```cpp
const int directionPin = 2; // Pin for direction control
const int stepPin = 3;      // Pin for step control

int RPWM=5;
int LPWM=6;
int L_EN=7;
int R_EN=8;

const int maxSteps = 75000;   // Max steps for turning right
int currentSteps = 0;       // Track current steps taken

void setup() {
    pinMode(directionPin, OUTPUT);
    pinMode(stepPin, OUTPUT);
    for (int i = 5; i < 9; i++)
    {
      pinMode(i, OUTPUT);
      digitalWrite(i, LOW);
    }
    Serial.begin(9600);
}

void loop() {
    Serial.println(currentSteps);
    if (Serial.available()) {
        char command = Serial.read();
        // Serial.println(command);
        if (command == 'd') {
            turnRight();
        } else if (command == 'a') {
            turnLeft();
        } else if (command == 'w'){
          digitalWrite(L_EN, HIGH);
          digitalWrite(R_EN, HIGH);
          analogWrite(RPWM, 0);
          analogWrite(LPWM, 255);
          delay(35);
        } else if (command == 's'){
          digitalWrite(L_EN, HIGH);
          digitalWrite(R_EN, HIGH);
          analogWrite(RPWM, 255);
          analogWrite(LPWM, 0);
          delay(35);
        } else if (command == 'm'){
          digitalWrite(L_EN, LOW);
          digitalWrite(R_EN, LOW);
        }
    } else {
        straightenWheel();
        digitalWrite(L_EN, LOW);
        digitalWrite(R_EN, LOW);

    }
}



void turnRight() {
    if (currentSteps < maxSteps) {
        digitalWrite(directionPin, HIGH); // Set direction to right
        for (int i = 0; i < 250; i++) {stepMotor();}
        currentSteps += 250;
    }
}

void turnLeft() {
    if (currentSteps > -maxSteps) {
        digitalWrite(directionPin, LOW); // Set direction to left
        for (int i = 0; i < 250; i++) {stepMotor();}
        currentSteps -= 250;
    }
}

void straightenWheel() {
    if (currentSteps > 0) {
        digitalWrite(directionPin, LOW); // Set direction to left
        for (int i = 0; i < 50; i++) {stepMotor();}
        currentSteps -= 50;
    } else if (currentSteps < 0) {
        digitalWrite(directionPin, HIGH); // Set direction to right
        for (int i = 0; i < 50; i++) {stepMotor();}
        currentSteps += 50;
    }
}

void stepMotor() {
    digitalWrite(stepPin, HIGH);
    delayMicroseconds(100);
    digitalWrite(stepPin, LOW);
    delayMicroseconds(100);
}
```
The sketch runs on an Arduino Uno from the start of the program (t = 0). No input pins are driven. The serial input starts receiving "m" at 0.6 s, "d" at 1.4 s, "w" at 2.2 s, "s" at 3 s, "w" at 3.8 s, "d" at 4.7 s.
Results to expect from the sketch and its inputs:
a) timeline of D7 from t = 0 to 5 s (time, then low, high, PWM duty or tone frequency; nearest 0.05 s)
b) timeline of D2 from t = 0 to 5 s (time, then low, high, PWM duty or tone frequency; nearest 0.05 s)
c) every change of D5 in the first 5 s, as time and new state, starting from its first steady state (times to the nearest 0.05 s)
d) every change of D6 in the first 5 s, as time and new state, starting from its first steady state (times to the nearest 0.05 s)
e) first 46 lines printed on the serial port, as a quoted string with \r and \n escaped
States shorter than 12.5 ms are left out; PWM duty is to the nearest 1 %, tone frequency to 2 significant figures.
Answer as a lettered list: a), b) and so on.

a) 0 s low; 2.2 s high; 2.25 s low; 3 s high; 3.05 s low; 3.8 s high; 3.85 s low
b) 0 s low; 1.4 s high; 1.45 s low; 4.7 s high; 4.75 s low
c) 0 s low; 3 s high; 3.8 s low
d) 0 s low; 2.2 s high; 3 s low; 3.8 s high
e) "0\r\n0\r\n0\r\n0\r\n0\r\n0\r\n0\r\n0\r\n0\r\n0\r\n0\r\n0\r\n0\r\n0\r\n0\r\n0\r\n0\r\n0\r\n0\r\n0\r\n0\r\n0\r\n0\r\n0\r\n0\r\n0\r\n0\r\n0\r\n0\r\n0\r\n0\r\n0\r\n0\r\n0\r\n0\r\n0\r\n0\r\n0\r\n0\r\n0\r\n0\r\n0\r\n0\r\n0\r\n0\r\n0\r\n"
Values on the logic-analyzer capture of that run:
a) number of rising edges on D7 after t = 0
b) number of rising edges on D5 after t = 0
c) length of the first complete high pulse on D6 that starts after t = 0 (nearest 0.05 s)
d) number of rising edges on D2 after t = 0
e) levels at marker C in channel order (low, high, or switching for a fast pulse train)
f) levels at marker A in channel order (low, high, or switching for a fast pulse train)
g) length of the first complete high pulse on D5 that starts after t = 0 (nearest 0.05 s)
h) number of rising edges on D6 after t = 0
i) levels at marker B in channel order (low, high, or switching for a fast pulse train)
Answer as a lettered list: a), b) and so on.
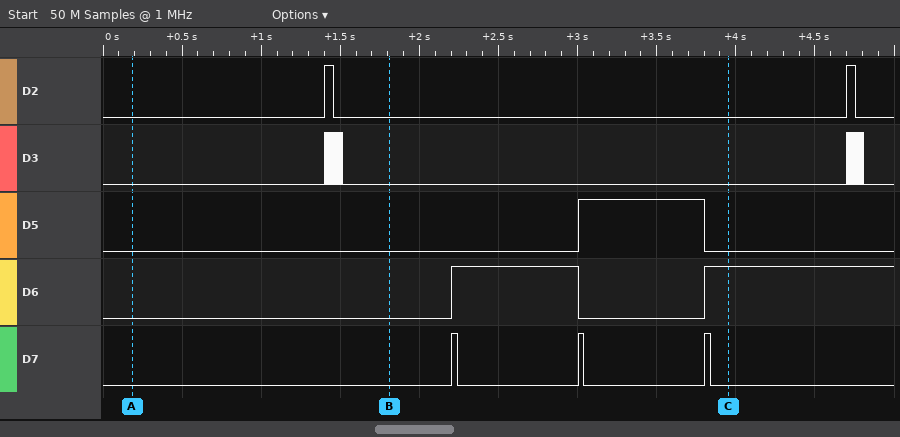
a) 3
b) 1
c) 0.80 s
d) 2
e) D2 low, D3 low, D5 low, D6 high, D7 low
f) D2 low, D3 low, D5 low, D6 low, D7 low
g) 0.80 s
h) 2
i) D2 low, D3 low, D5 low, D6 low, D7 low
